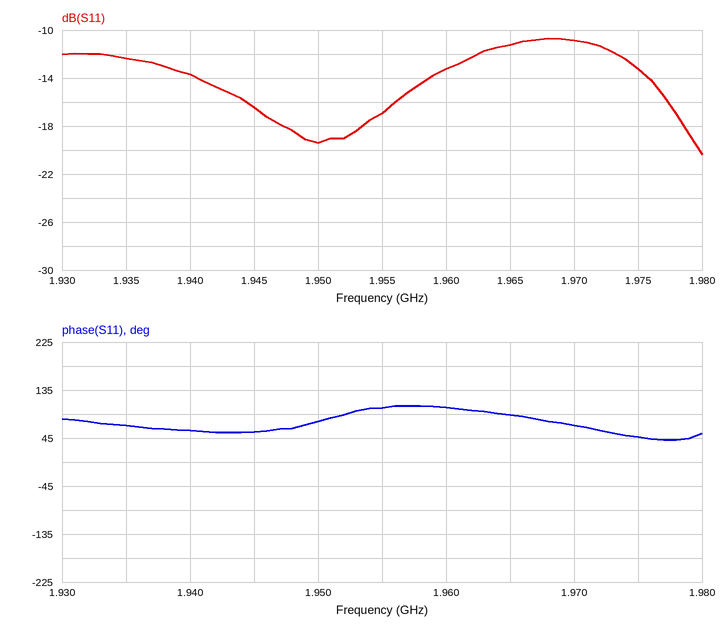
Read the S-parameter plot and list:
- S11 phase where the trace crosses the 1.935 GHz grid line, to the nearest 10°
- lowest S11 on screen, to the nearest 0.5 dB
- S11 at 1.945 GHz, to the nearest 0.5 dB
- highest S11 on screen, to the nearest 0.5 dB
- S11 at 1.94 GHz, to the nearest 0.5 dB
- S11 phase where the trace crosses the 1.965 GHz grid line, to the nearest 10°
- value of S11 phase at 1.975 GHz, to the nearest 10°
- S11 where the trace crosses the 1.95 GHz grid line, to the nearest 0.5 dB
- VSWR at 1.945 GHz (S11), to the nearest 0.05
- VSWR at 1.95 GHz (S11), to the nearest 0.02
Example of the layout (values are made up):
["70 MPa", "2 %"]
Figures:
["70°", "-20.5 dB", "-16.5 dB", "-10.5 dB", "-13.5 dB", "90°", "50°", "-19.5 dB", "1.35", "1.24"]
